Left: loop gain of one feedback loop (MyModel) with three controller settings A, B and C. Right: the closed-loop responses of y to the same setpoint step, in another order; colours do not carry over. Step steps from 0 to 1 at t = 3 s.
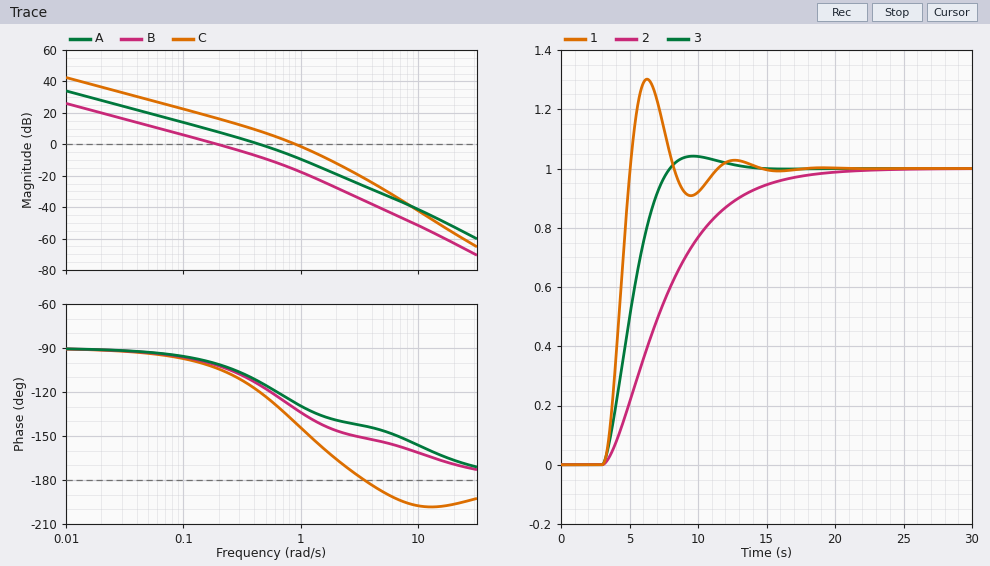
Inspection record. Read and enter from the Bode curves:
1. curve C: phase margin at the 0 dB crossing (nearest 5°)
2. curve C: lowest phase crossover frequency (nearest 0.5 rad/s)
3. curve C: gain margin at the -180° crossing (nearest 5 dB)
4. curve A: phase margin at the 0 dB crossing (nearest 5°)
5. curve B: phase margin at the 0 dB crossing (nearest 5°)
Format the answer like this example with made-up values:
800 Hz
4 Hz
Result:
40°
3.5 rad/s
20 dB
65°
80°
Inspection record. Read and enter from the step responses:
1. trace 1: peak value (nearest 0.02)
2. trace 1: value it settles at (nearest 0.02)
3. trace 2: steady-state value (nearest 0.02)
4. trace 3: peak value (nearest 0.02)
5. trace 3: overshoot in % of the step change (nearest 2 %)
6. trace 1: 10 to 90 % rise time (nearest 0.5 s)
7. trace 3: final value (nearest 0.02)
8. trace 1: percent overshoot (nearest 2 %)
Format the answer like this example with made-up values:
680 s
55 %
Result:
1.30
1.00
1.00
1.04
4 %
1.5 s
1.00
30 %
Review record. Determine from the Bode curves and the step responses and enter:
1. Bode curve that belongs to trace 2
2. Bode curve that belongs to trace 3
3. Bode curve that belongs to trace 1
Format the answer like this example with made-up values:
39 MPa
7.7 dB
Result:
B
A
C
